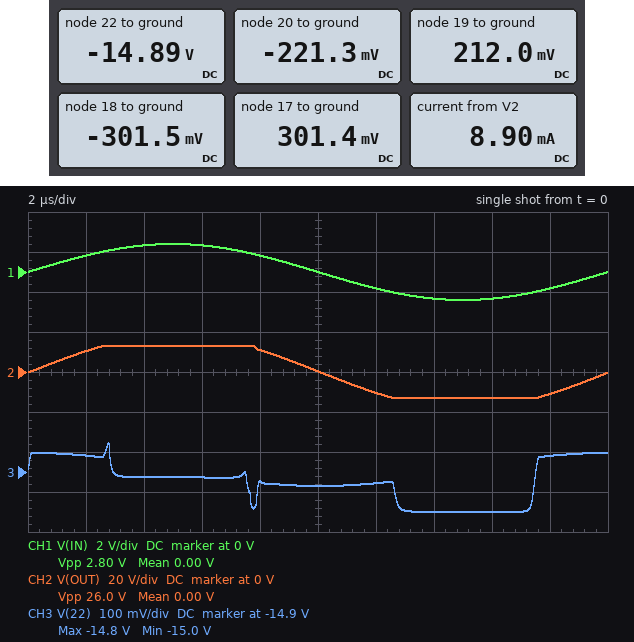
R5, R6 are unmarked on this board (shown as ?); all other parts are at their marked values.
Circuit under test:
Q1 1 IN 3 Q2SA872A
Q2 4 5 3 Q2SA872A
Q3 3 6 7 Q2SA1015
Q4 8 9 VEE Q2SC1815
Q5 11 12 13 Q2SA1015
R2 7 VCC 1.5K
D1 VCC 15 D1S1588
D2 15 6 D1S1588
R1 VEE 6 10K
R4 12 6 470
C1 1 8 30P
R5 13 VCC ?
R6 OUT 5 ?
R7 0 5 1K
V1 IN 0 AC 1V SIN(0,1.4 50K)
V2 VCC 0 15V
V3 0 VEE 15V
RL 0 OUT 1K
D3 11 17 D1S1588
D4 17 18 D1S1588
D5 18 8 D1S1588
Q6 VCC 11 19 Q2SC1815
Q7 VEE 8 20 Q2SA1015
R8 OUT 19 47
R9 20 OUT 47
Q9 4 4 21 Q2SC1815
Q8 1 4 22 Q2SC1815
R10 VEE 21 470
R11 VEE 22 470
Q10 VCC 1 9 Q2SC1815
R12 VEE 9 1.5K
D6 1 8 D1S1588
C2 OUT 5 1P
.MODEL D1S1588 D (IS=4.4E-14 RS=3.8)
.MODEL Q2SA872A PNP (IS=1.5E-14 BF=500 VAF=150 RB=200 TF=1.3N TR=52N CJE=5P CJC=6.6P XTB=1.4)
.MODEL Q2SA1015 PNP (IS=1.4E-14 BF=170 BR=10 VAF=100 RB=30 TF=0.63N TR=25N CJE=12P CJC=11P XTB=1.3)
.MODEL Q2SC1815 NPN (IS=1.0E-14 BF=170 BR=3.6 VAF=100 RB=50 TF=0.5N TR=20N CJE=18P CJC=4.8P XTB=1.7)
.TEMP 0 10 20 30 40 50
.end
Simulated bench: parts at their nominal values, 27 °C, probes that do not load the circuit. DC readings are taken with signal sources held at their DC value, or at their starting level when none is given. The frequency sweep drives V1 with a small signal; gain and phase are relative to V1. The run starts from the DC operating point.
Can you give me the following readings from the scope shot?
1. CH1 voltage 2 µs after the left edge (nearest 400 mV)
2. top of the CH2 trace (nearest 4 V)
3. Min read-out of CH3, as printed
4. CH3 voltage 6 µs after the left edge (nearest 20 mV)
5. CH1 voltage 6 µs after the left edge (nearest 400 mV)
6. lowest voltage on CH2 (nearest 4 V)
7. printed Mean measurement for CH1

800 mV
12 V
-15.0 V
-14.92 V
1.2 V
-12 V
0.00 V
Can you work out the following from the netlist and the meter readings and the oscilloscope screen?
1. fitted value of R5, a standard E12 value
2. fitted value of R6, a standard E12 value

1.2 kΩ
12 kΩ
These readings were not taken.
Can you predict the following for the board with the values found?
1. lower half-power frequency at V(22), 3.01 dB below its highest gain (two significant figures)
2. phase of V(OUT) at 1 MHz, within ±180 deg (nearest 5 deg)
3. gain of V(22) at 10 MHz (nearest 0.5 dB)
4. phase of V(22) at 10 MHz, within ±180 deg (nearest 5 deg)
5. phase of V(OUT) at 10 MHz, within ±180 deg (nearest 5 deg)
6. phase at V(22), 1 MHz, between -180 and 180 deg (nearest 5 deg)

2.3 MHz
-20 deg
1.5 dB
-55 deg
-155 deg
70 deg
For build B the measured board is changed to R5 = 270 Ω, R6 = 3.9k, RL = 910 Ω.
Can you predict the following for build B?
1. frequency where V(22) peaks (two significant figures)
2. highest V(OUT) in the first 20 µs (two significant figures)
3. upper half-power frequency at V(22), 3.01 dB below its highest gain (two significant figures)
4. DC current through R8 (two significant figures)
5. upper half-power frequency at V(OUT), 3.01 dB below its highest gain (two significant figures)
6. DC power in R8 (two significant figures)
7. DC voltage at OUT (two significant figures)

7.7 MHz
6.9 V
11 MHz
5.9 mA
9.2 MHz
1.6 mW
-1.3 mV
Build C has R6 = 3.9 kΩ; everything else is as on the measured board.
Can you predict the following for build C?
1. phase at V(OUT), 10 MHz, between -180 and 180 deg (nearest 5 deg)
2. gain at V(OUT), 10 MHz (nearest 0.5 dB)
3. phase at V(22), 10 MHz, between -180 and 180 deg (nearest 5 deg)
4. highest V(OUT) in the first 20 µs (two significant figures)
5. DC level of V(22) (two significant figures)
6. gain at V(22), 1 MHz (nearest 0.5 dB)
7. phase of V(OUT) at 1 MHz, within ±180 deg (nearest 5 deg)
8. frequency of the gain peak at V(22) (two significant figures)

-145 deg
13.0 dB
-45 deg
6.9 V
-15 V
-13.0 dB
-5 deg
7.6 MHz
